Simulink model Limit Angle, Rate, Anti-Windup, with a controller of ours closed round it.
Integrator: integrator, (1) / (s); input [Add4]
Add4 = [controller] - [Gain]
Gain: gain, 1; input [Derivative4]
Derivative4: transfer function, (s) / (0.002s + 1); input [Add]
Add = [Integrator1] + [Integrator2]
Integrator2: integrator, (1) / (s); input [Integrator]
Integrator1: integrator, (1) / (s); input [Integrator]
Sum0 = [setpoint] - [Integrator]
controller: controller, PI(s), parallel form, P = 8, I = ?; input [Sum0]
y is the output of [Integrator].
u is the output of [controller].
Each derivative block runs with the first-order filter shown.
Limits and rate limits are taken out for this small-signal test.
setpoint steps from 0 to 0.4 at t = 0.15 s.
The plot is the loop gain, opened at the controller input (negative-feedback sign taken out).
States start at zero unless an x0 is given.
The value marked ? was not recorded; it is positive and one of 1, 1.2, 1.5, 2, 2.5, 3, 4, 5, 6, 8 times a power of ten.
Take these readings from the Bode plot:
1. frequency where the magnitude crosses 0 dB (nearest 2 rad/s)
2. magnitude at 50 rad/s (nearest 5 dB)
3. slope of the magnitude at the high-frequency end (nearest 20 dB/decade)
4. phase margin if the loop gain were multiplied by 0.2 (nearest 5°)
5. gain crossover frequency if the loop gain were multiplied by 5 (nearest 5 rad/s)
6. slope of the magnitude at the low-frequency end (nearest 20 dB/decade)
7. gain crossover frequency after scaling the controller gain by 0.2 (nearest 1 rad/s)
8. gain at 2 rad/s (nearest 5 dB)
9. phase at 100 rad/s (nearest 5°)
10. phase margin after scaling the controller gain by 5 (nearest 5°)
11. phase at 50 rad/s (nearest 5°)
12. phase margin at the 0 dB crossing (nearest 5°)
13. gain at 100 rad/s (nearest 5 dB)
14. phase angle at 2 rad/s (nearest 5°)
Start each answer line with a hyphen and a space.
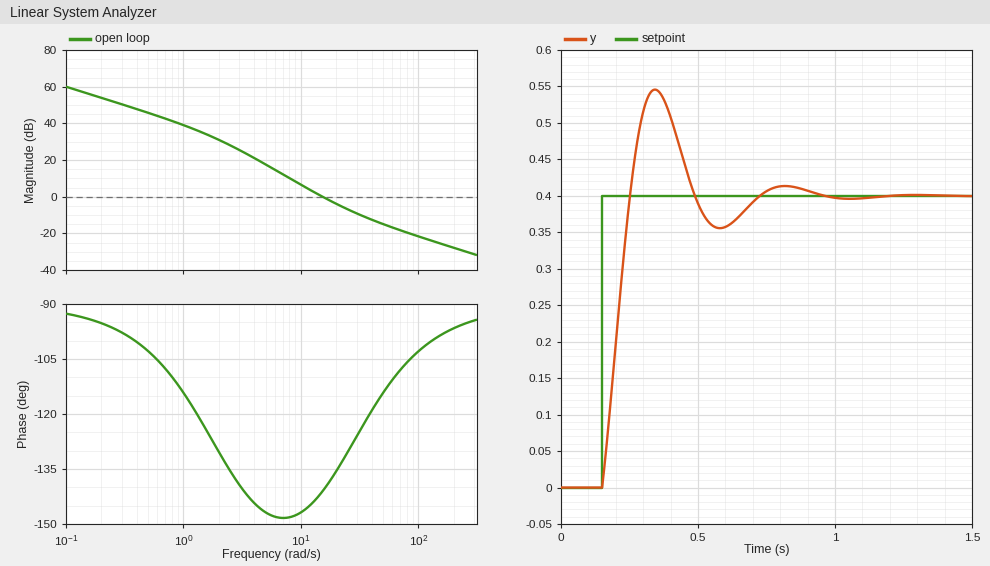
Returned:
- 16 rad/s
- -15 dB
- -20 dB/decade
- 30°
- 45 rad/s
- -20 dB/decade
- 6 rad/s
- 30 dB
- -105°
- 65°
- -115°
- 40°
- -20 dB
- -130°
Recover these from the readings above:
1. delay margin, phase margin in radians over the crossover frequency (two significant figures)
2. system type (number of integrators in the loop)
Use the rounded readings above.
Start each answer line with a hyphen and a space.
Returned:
- 0.044 s
- 1
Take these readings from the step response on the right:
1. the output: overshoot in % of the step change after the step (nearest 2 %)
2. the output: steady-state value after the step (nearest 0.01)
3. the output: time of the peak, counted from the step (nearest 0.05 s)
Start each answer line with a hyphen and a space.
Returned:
- 36 %
- 0.40
- 0.20 s
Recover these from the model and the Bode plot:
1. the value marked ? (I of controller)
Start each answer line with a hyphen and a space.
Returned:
- 200
